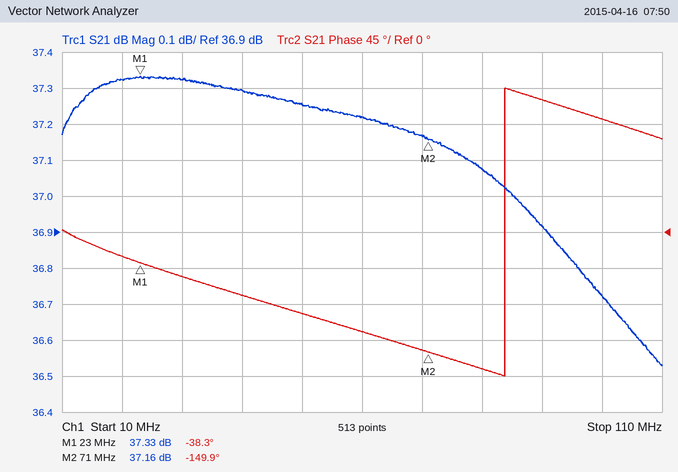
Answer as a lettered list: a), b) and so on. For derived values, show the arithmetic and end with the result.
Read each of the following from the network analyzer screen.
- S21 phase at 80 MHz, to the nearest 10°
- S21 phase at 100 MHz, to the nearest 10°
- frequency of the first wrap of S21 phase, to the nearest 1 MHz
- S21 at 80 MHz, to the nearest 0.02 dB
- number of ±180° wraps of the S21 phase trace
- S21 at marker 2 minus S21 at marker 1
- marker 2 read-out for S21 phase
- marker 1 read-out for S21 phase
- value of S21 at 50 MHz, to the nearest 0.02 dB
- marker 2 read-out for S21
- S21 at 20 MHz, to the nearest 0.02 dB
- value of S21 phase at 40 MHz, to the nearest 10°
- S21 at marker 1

a) -170°
b) 140°
c) 84 MHz
d) 37.08 dB
e) 1
f) 37.16 − (37.33) = -0.17 dB
g) -149.9°
h) -38.3°
i) 37.26 dB
j) 37.16 dB
k) 37.32 dB
l) -80°
m) 37.33 dB
